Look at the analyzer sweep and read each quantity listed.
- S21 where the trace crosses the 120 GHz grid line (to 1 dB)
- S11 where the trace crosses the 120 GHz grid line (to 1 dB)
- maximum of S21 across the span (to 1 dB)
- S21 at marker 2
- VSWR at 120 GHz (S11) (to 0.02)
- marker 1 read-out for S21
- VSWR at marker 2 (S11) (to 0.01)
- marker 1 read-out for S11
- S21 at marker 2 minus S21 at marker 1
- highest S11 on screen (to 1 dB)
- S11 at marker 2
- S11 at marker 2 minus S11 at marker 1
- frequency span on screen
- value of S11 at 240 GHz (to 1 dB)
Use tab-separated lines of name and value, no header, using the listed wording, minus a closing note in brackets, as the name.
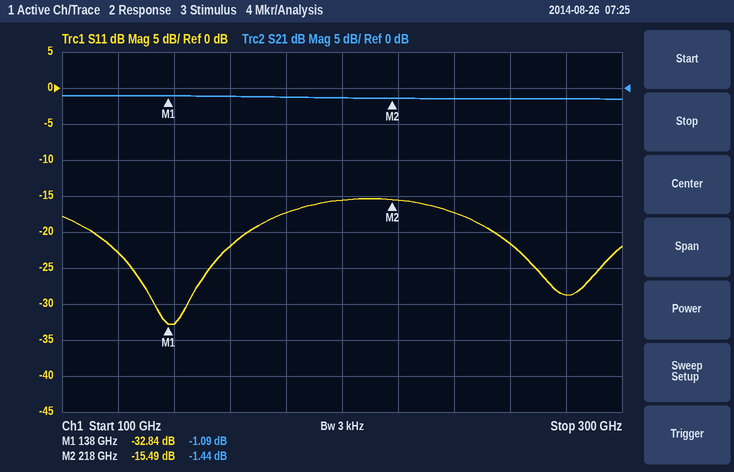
S21 where the trace crosses the 120 GHz grid line	-1 dB
S11 where the trace crosses the 120 GHz grid line	-23 dB
maximum of S21 across the span	-1 dB
S21 at marker 2	-1.44 dB
VSWR at 120 GHz (S11)	1.16
marker 1 read-out for S21	-1.09 dB
VSWR at marker 2 (S11)	1.40
marker 1 read-out for S11	-32.84 dB
S21 at marker 2 minus S21 at marker 1	-0.35 dB
highest S11 on screen	-15 dB
S11 at marker 2	-15.49 dB
S11 at marker 2 minus S11 at marker 1	17.35 dB
frequency span on screen	200 GHz
value of S11 at 240 GHz	-17 dB
